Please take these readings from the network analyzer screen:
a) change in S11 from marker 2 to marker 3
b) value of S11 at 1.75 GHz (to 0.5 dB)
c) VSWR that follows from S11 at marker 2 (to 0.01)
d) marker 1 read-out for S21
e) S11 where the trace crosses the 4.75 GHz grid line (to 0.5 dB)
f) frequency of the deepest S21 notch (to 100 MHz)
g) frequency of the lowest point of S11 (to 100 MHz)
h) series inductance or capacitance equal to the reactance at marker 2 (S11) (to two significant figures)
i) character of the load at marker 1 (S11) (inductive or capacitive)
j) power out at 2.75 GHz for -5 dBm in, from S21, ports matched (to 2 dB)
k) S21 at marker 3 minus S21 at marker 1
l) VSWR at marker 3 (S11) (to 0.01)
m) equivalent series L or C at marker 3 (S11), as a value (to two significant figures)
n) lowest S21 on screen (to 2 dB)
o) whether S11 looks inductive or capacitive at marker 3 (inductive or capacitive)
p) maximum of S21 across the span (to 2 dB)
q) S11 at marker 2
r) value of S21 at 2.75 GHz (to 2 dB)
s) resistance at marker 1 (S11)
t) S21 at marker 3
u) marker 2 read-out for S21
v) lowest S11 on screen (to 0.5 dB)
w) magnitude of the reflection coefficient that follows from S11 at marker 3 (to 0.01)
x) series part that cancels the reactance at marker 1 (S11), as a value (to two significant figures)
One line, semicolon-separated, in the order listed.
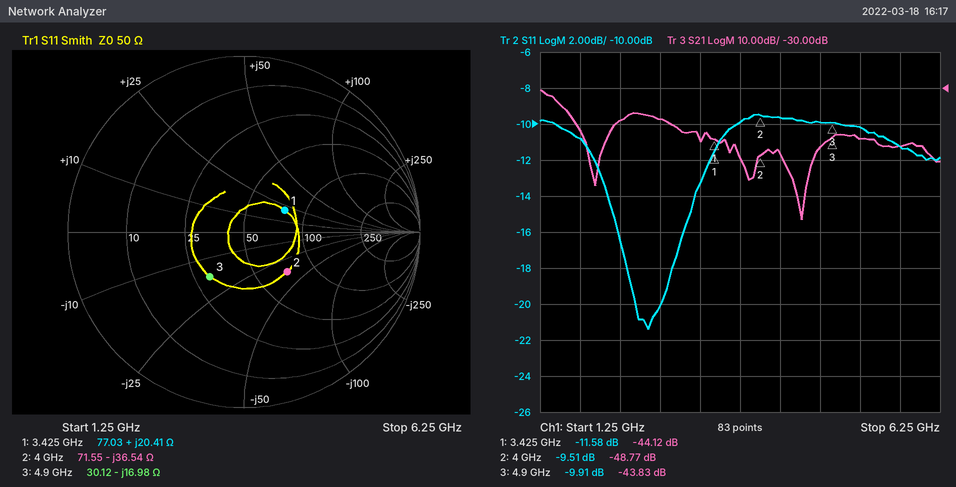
-0.40 dB; -11.0 dB; 2.01; -44.12 dB; -10.0 dB; 4.5 GHz; 2.6 GHz; 1.1 pF; inductive; -44 dBm; 0.29 dB; 1.94; 1.9 pF; -66 dB; capacitive; -30 dB; -9.51 dB; -38 dB; 77.03 Ω; -43.83 dB; -48.77 dB; -21.5 dB; 0.32; 2.3 pF
